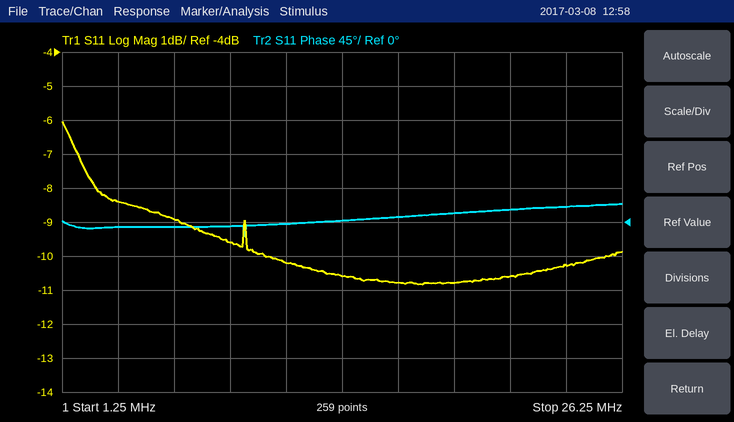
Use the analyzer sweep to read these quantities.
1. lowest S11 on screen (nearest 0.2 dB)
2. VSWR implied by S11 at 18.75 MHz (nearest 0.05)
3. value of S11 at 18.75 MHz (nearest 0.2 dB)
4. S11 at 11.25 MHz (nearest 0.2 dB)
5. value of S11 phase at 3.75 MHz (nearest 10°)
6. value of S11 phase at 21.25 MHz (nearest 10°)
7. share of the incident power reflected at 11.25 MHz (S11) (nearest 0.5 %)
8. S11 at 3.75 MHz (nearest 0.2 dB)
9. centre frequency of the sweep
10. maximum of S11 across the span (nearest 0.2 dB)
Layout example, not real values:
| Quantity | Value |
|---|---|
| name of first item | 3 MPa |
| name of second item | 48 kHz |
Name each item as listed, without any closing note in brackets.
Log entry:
| Quantity | Value |
|---|---|
| lowest S11 on screen | -10.8 dB |
| VSWR implied by S11 at 18.75 MHz | 1.80 |
| value of S11 at 18.75 MHz | -10.8 dB |
| S11 at 11.25 MHz | -10.2 dB |
| value of S11 phase at 3.75 MHz | -10° |
| value of S11 phase at 21.25 MHz | 20° |
| share of the incident power reflected at 11.25 MHz (S11) | 9.5 % |
| S11 at 3.75 MHz | -8.4 dB |
| centre frequency of the sweep | 13.75 MHz |
| maximum of S11 across the span | -6.0 dB |
